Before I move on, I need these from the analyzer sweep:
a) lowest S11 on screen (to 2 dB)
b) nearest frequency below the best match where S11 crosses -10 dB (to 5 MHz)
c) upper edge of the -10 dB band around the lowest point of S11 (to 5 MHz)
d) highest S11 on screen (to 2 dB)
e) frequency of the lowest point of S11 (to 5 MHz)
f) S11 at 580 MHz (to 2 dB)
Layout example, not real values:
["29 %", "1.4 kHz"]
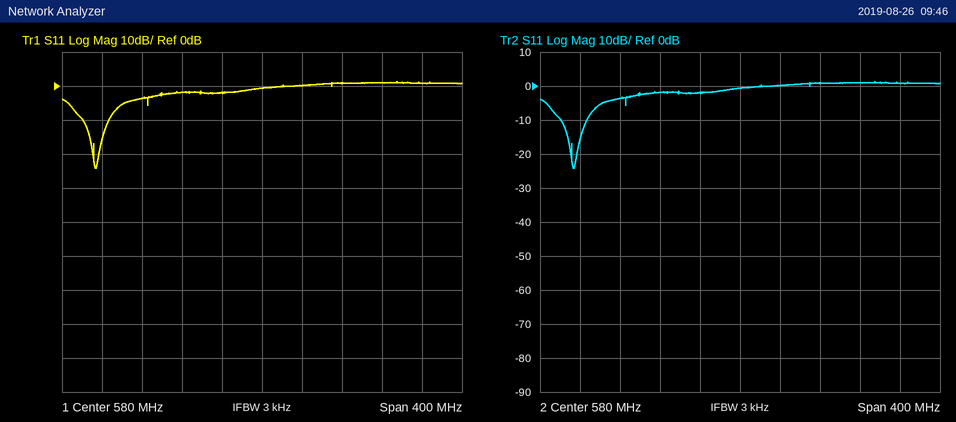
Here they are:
["-24 dB", "400 MHz", "425 MHz", "2 dB", "415 MHz", "0 dB"]
